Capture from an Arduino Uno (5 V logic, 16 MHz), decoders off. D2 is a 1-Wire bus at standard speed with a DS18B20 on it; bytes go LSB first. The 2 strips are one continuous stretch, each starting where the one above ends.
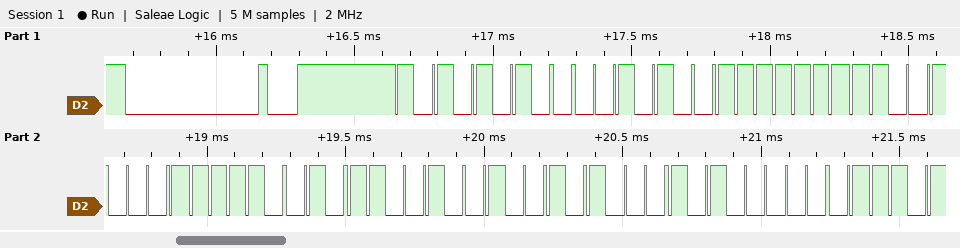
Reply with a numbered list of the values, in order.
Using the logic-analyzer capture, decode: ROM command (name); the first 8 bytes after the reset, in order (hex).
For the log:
1. Match ROM
2. 55 28 FF 89 4F 93 14 05
